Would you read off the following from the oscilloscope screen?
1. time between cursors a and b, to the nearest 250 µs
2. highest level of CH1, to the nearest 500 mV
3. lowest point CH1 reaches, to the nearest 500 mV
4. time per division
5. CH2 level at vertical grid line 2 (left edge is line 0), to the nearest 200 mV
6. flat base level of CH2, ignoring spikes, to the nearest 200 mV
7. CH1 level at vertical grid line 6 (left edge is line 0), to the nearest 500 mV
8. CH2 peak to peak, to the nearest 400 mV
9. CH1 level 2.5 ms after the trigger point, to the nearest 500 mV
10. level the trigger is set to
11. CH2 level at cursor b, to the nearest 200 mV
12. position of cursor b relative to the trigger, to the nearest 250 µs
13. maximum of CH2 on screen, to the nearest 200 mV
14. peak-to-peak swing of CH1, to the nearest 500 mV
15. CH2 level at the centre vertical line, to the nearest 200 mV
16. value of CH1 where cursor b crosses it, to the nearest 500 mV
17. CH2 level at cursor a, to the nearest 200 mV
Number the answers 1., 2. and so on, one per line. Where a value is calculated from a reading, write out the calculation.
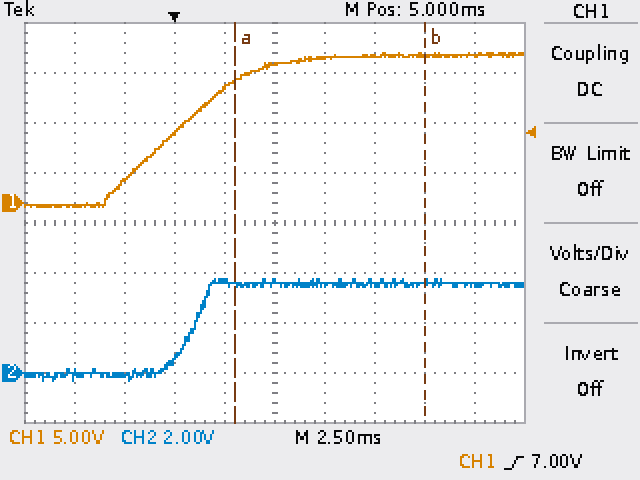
1. 9.50 ms
2. 15.0 V
3. -500 mV
4. 2.5 ms
5. 0.0 V
6. 0.0 V
7. 14.5 V
8. 4.0 V
9. 11.5 V
10. 7.00 V
11. 3.6 V
12. +12.50 ms
13. 3.8 V
14. 15.0 V − (-500 mV) = 15.5 V
15. 3.6 V
16. 15.0 V
17. 3.6 V
